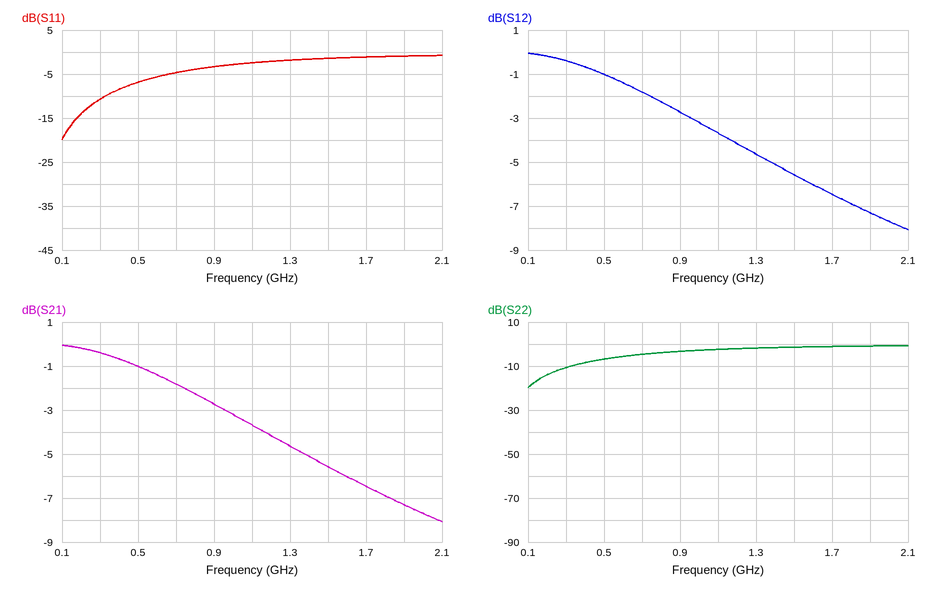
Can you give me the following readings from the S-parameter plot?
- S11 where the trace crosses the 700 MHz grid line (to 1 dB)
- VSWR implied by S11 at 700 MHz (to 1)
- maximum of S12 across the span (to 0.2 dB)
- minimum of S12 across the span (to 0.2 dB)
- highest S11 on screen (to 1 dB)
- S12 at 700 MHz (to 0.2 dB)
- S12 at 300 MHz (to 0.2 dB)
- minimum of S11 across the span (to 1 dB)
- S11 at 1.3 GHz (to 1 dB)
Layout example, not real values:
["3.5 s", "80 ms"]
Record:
["-5 dB", "4", "0.0 dB", "-8.0 dB", "-1 dB", "-1.8 dB", "-0.4 dB", "-20 dB", "-2 dB"]
